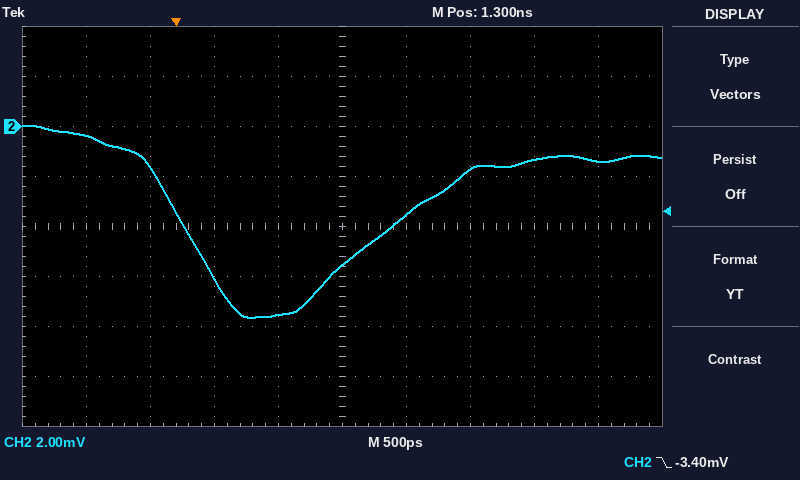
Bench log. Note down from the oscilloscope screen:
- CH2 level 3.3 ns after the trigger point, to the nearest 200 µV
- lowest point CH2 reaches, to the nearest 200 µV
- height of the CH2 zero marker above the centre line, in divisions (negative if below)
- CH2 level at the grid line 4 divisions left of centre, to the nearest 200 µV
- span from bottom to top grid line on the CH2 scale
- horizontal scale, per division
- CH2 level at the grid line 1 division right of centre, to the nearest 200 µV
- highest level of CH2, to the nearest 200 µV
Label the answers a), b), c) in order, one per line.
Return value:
a) -1.4 mV
b) -7.6 mV
c) +2.0 div
d) -400 µV
e) 16 mV
f) 500 ps
g) -3.6 mV
h) 0.0 mV
